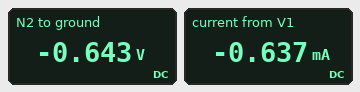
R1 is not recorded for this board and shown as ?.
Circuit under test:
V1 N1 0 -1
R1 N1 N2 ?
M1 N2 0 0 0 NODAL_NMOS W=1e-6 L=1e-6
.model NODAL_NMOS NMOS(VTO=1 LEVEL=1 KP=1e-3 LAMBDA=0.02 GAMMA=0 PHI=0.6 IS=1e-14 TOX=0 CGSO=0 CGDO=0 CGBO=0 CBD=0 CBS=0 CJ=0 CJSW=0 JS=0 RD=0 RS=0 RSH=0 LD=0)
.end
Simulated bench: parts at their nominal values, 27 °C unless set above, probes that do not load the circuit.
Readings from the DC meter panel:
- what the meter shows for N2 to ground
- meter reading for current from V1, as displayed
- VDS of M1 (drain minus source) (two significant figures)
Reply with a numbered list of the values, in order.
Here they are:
1. -0.643 V
2. -0.637 mA
3. -640 mV
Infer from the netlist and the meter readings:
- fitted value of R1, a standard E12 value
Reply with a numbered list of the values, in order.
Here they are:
1. 560 Ω
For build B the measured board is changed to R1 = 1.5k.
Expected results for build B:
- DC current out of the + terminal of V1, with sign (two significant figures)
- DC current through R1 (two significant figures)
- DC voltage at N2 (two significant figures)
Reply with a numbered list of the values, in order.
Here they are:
1. -250 µA
2. 250 µA
3. -620 mV
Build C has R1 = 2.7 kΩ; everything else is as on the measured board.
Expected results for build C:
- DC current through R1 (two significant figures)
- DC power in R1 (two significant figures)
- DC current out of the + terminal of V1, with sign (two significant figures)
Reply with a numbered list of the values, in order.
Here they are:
1. 150 µA
2. 58 µW
3. -150 µA
